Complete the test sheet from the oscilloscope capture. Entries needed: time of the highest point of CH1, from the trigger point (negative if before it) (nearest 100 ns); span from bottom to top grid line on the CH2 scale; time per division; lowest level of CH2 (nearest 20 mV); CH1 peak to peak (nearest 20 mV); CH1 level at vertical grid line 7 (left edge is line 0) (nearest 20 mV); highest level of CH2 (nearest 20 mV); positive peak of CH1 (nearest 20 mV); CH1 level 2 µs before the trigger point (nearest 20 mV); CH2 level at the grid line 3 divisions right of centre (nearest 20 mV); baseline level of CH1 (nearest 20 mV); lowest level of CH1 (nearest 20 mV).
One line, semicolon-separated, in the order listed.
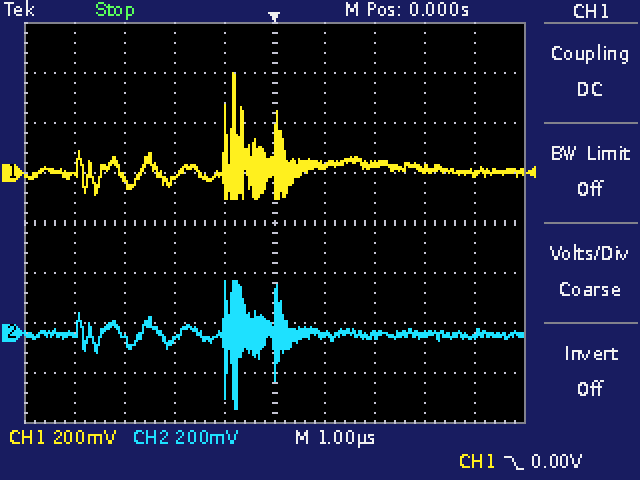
-800 ns; 1.6 V; 1 µs; -300 mV; 500 mV; 40 mV; 200 mV; 400 mV; -20 mV; 0 mV; 20 mV; -100 mV
